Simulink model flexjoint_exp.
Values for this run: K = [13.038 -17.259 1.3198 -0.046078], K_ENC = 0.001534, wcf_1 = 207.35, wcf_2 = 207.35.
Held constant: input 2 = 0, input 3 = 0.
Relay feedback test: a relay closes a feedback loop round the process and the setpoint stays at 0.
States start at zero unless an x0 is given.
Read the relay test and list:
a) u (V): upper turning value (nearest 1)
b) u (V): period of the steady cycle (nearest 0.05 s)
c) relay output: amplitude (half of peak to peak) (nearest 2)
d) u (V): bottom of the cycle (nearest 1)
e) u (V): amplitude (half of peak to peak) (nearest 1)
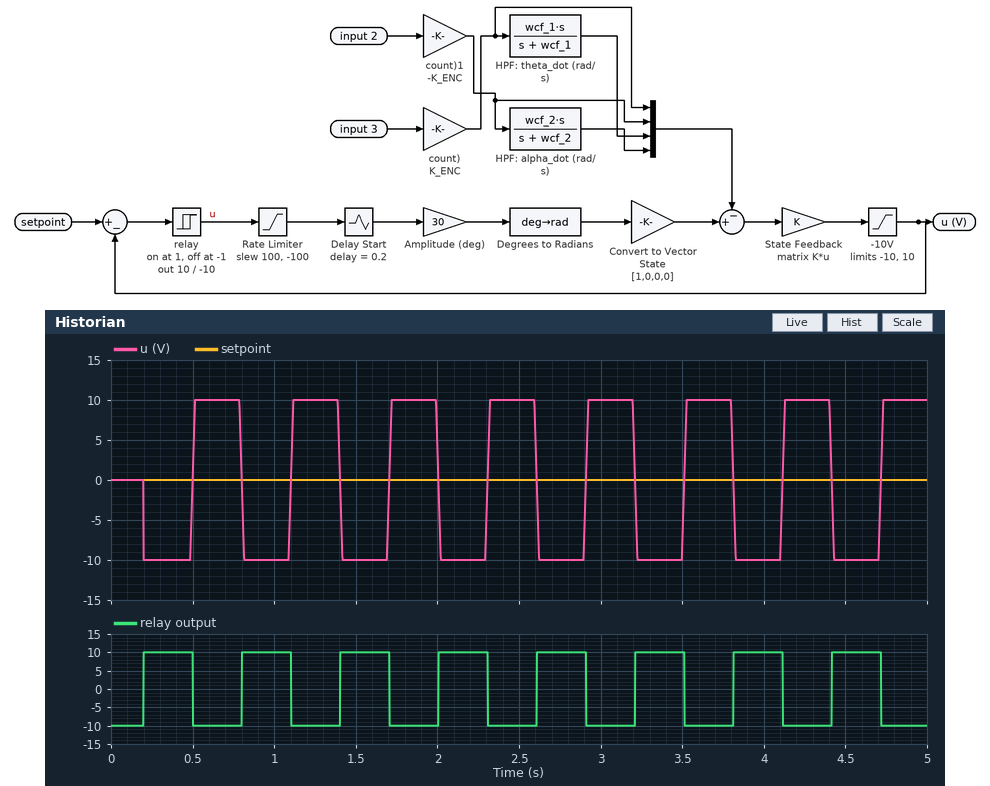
10
0.60 s
10
-10
10
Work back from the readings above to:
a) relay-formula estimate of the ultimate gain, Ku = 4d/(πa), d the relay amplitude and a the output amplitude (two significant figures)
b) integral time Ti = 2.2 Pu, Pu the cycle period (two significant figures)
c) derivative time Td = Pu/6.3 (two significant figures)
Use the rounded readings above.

1.3
1.3 s
0.095 s
